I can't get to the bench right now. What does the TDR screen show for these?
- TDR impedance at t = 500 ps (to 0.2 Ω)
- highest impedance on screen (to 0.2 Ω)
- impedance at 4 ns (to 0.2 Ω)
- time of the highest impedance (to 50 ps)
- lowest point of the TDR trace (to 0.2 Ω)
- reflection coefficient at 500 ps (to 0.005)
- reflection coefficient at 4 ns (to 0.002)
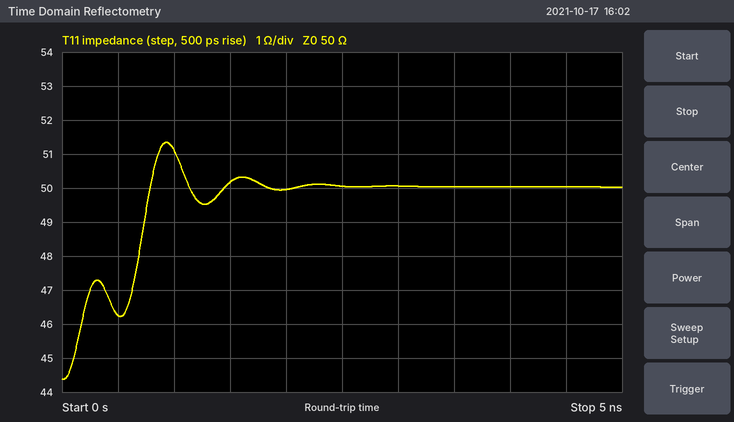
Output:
46.2 Ω
51.4 Ω
50.0 Ω
950 ps
44.4 Ω
-0.040
0.000
